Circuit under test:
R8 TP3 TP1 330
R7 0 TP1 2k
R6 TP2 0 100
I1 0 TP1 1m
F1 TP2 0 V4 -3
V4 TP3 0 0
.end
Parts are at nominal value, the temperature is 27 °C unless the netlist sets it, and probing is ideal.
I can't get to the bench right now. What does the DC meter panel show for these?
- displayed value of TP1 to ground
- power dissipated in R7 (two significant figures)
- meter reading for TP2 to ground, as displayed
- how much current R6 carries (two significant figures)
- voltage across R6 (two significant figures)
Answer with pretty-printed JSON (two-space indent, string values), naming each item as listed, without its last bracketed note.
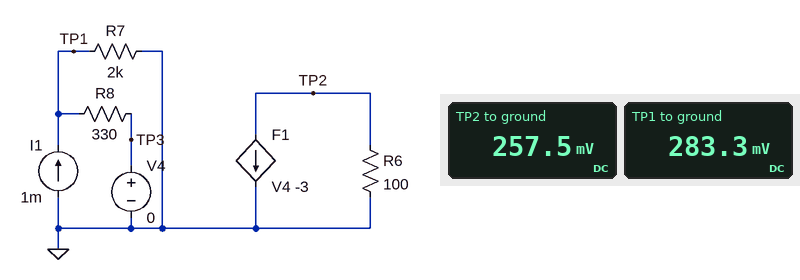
{
  "displayed value of TP1 to ground": "283.3 mV",
  "power dissipated in R7": "40 µW",
  "meter reading for TP2 to ground, as displayed": "257.5 mV",
  "how much current R6 carries": "2.6 mA",
  "voltage across R6": "260 mV"
}
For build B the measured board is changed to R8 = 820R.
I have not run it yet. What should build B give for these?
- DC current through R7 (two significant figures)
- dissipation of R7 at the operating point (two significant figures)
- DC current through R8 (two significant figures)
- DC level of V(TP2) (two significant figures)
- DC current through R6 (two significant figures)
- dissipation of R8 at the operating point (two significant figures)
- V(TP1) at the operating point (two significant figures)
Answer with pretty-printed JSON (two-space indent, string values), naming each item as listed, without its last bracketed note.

{
  "DC current through R7": "290 µA",
  "dissipation of R7 at the operating point": "170 µW",
  "DC current through R8": "710 µA",
  "DC level of V(TP2)": "210 mV",
  "DC current through R6": "2.1 mA",
  "dissipation of R8 at the operating point": "410 µW",
  "V(TP1) at the operating point": "580 mV"
}
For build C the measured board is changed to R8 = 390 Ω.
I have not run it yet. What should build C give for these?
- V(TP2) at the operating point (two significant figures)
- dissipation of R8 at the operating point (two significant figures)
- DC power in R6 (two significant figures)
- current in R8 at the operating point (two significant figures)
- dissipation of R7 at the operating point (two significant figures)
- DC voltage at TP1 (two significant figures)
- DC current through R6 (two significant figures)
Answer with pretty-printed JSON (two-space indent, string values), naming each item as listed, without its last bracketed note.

{
  "V(TP2) at the operating point": "250 mV",
  "dissipation of R8 at the operating point": "270 µW",
  "DC power in R6": "630 µW",
  "current in R8 at the operating point": "840 µA",
  "dissipation of R7 at the operating point": "53 µW",
  "DC voltage at TP1": "330 mV",
  "DC current through R6": "2.5 mA"
}
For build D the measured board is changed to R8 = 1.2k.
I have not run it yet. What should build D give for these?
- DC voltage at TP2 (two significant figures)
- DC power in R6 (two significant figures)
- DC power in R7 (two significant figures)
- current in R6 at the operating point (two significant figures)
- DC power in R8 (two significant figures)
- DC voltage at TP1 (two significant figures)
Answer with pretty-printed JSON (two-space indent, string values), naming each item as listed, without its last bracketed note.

{
  "DC voltage at TP2": "190 mV",
  "DC power in R6": "350 µW",
  "DC power in R7": "280 µW",
  "current in R6 at the operating point": "1.9 mA",
  "DC power in R8": "470 µW",
  "DC voltage at TP1": "750 mV"
}
